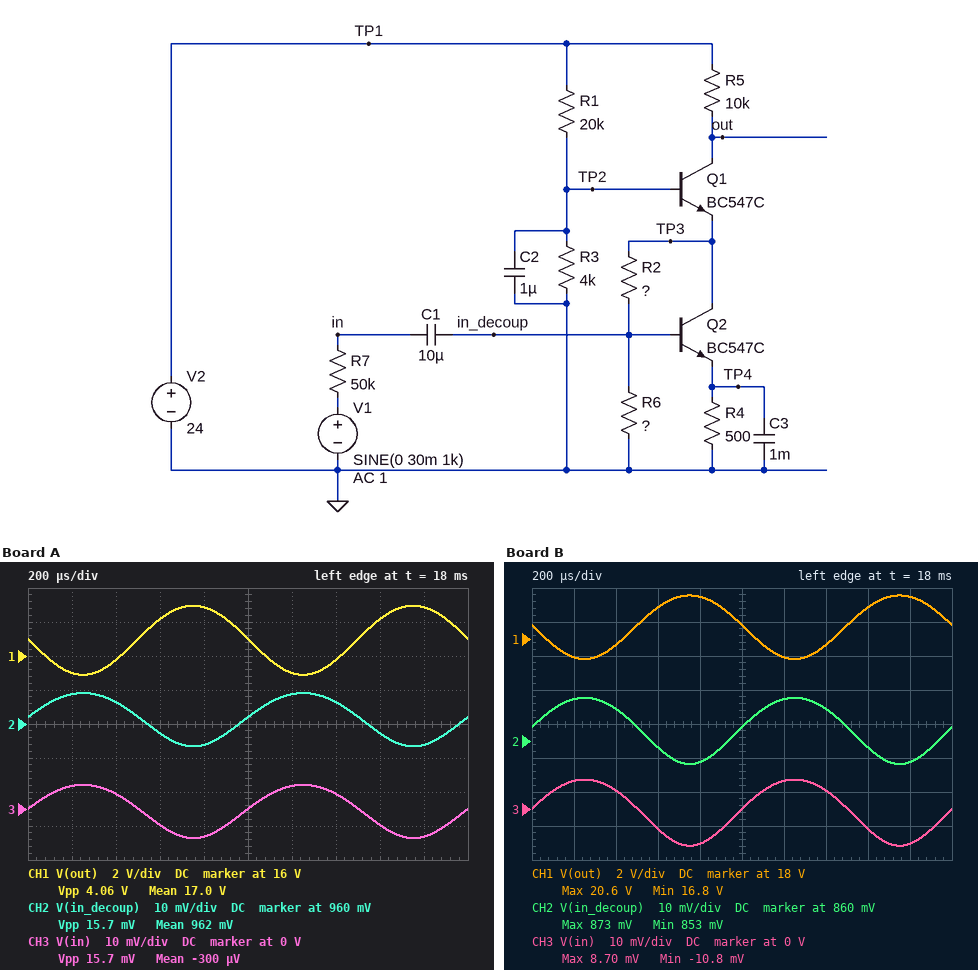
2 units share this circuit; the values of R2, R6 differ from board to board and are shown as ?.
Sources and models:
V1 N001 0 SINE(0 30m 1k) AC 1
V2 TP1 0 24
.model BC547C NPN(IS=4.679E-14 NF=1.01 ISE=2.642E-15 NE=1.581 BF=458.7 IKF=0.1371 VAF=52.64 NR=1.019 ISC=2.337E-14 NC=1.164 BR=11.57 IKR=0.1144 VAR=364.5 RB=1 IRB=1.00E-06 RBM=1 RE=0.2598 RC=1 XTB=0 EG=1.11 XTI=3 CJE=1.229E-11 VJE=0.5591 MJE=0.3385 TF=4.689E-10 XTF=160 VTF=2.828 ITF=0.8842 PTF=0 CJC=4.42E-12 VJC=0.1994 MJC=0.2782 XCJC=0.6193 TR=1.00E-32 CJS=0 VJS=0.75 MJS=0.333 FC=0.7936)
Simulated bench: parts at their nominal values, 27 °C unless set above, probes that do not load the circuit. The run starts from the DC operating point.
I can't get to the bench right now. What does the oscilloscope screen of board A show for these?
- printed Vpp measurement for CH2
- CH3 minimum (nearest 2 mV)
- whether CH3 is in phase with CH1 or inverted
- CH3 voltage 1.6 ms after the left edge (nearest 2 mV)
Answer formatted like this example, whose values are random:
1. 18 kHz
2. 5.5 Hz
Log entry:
1. 15.7 mV
2. -8 mV
3. inverted
4. -4 mV
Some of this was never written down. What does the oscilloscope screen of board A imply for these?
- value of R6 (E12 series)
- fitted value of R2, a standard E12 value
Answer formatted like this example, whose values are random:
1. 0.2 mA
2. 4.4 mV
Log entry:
1. 6.8 MΩ
2. 1.5 MΩ
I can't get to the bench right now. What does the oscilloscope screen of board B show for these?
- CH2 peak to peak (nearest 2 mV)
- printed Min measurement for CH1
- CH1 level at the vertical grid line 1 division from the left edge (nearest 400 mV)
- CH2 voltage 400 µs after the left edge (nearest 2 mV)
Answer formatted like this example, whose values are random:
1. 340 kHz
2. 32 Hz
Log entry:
1. 20 mV
2. 16.8 V
3. 16.8 V
4. 870 mV
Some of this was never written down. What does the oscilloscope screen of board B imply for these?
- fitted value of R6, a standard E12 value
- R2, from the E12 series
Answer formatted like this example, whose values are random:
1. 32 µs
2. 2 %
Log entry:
1. 15 MΩ
2. 2.2 MΩ
